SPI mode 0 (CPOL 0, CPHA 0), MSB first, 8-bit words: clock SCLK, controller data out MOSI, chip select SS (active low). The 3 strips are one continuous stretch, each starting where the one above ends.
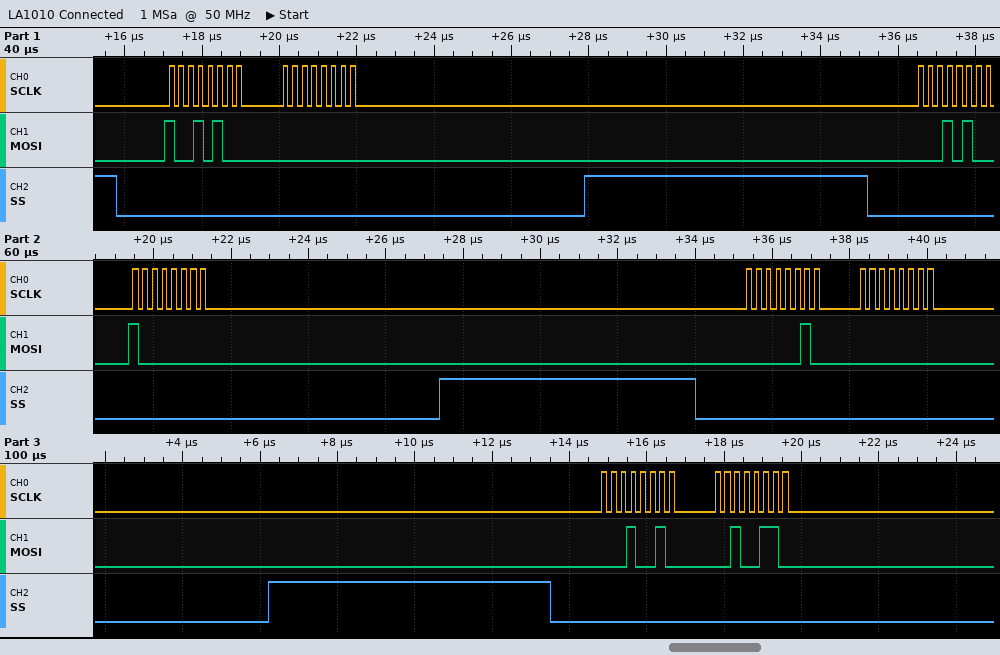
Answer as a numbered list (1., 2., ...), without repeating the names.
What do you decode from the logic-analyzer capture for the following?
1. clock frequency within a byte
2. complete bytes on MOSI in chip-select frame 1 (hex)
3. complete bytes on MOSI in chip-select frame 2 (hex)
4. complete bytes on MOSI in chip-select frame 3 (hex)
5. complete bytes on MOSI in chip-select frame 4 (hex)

1. 4 MHz
2. 94 00
3. 14 80
4. 02 00
5. 12 26
